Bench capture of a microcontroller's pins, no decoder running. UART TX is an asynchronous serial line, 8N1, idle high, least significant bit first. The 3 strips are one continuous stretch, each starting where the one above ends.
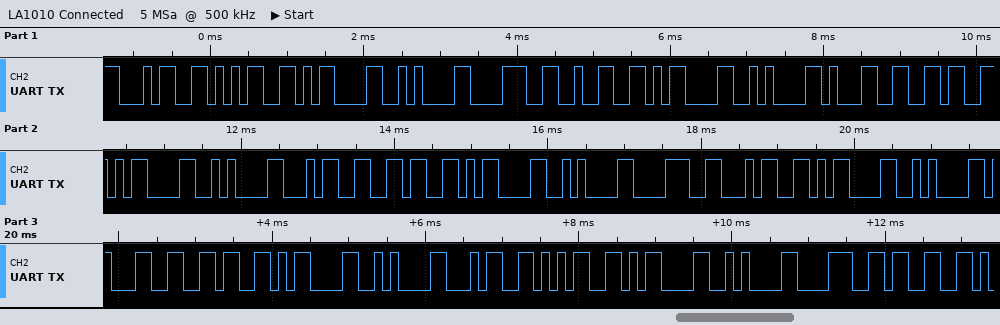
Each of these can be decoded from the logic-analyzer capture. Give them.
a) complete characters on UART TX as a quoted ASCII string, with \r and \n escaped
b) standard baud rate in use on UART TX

"45\r\n82\r\n16\r\n46\r\n84\r\n16\r\n45\r\n83"
9600 baud
